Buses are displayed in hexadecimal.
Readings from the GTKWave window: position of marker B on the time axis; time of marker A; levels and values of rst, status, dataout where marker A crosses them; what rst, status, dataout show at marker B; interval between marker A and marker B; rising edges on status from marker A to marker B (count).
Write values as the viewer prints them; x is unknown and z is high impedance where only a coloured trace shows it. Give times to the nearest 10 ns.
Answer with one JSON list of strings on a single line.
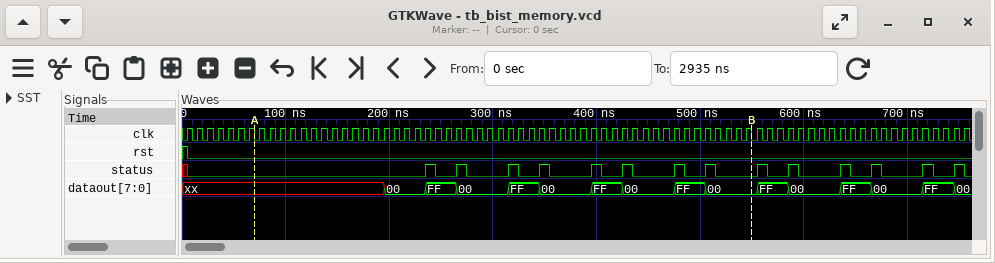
["550 ns", "70 ns", "rst=0, status=0, dataout=xx", "rst=0, status=0, dataout=00", "480 ns", "8"]
